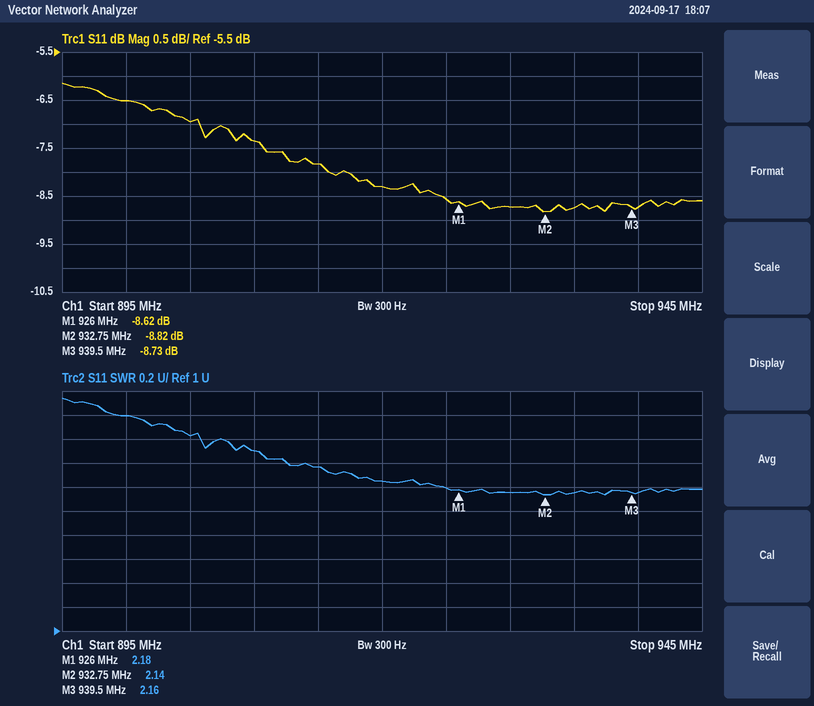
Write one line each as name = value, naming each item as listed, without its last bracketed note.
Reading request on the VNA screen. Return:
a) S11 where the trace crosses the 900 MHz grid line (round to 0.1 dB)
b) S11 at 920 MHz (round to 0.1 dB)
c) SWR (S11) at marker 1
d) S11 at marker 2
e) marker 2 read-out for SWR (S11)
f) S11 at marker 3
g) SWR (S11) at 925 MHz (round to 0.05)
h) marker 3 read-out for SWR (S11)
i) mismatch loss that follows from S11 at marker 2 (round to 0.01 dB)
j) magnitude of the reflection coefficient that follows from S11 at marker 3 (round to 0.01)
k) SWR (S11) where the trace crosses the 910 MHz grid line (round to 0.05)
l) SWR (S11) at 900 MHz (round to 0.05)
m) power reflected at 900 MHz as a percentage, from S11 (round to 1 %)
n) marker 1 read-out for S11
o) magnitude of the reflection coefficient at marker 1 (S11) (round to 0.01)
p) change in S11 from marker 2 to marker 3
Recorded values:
S11 where the trace crosses the 900 MHz grid line = -6.5 dB
S11 at 920 MHz = -8.3 dB
SWR (S11) at marker 1 = 2.18
S11 at marker 2 = -8.82 dB
marker 2 read-out for SWR = 2.14
S11 at marker 3 = -8.73 dB
SWR (S11) at 925 MHz = 2.20
marker 3 read-out for SWR = 2.16
mismatch loss that follows from S11 at marker 2 = 0.61 dB
magnitude of the reflection coefficient that follows from S11 at marker 3 = 0.37
SWR (S11) where the trace crosses the 910 MHz grid line = 2.50
SWR (S11) at 900 MHz = 2.80
power reflected at 900 MHz as a percentage, from S11 = 22 %
marker 1 read-out for S11 = -8.62 dB
magnitude of the reflection coefficient at marker 1 (S11) = 0.37
change in S11 from marker 2 to marker 3 = 0.09 dB
